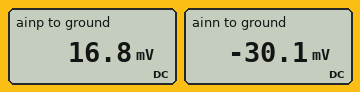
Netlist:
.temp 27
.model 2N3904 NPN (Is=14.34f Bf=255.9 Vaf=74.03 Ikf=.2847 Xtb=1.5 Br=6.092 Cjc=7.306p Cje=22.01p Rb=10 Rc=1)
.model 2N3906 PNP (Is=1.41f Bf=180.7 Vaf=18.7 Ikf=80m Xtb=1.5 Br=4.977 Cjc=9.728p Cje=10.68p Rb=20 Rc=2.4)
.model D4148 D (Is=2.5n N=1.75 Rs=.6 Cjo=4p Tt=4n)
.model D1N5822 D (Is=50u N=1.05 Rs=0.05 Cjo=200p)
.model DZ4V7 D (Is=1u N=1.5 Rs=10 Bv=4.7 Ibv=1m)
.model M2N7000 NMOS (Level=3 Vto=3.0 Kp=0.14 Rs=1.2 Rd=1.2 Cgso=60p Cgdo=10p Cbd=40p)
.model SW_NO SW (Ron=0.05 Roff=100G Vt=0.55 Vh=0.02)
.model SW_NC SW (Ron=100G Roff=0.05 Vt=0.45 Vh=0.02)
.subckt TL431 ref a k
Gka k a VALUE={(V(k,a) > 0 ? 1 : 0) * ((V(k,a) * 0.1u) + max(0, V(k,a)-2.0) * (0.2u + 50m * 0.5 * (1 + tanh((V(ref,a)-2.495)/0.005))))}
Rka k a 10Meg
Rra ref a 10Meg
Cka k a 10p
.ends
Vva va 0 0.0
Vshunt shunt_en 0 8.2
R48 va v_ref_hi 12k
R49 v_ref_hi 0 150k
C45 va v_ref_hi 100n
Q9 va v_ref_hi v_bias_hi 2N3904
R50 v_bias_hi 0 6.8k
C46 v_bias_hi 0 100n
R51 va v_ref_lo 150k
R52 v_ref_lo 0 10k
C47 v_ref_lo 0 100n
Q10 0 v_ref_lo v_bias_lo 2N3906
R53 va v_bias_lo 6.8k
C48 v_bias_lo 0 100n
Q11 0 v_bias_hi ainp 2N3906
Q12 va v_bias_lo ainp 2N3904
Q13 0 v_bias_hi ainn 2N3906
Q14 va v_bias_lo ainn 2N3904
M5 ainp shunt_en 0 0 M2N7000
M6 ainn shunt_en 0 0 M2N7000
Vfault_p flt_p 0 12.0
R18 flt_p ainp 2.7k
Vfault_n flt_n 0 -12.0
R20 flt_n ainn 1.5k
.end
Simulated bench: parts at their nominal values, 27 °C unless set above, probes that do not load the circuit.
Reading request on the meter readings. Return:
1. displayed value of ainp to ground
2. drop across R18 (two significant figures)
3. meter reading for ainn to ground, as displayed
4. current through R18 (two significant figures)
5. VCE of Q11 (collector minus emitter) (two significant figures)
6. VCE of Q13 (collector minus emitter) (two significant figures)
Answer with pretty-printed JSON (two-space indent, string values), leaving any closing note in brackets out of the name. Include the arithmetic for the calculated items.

{
  "displayed value of ainp to ground": "16.8 mV",
  "drop across R18": "12 V - 16.8 mV = 12 V",
  "meter reading for ainn to ground, as displayed": "-30.1 mV",
  "current through R18": "(12 V - 16.8 mV) / 2.7 kΩ = 4.4 mA",
  "VCE of Q11 (collector minus emitter)": "0 V - 16.8 mV = -17 mV",
  "VCE of Q13 (collector minus emitter)": "0 V - (-30.1 mV) = 30 mV"
}
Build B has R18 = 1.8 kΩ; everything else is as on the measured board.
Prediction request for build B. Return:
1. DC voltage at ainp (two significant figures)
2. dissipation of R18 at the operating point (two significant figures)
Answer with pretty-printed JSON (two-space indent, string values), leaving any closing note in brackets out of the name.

{
  "DC voltage at ainp": "25 mV",
  "dissipation of R18 at the operating point": "80 mW"
}
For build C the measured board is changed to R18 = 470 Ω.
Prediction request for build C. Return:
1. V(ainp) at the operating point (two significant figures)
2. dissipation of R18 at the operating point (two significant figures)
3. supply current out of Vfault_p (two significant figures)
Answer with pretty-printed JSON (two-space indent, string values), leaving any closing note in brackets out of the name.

{
  "V(ainp) at the operating point": "96 mV",
  "dissipation of R18 at the operating point": "300 mW",
  "supply current out of Vfault_p": "25 mA"
}
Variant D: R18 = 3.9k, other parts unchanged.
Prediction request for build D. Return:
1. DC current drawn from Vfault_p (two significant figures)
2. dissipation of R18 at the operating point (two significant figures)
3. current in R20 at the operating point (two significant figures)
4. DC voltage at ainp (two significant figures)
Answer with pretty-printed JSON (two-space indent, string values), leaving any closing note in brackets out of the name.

{
  "DC current drawn from Vfault_p": "3.1 mA",
  "dissipation of R18 at the operating point": "37 mW",
  "current in R20 at the operating point": "8.0 mA",
  "DC voltage at ainp": "12 mV"
}
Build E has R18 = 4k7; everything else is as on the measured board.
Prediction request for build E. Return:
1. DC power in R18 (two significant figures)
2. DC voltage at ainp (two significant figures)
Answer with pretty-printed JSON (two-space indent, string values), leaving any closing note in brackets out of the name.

{
  "DC power in R18": "31 mW",
  "DC voltage at ainp": "9.6 mV"
}
